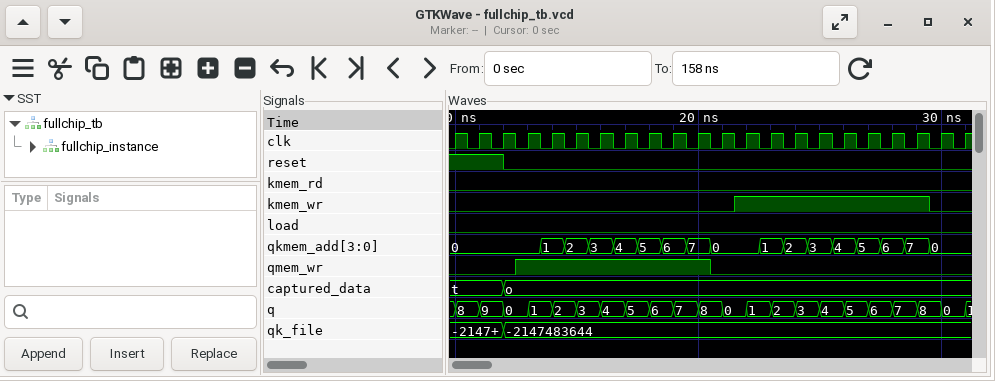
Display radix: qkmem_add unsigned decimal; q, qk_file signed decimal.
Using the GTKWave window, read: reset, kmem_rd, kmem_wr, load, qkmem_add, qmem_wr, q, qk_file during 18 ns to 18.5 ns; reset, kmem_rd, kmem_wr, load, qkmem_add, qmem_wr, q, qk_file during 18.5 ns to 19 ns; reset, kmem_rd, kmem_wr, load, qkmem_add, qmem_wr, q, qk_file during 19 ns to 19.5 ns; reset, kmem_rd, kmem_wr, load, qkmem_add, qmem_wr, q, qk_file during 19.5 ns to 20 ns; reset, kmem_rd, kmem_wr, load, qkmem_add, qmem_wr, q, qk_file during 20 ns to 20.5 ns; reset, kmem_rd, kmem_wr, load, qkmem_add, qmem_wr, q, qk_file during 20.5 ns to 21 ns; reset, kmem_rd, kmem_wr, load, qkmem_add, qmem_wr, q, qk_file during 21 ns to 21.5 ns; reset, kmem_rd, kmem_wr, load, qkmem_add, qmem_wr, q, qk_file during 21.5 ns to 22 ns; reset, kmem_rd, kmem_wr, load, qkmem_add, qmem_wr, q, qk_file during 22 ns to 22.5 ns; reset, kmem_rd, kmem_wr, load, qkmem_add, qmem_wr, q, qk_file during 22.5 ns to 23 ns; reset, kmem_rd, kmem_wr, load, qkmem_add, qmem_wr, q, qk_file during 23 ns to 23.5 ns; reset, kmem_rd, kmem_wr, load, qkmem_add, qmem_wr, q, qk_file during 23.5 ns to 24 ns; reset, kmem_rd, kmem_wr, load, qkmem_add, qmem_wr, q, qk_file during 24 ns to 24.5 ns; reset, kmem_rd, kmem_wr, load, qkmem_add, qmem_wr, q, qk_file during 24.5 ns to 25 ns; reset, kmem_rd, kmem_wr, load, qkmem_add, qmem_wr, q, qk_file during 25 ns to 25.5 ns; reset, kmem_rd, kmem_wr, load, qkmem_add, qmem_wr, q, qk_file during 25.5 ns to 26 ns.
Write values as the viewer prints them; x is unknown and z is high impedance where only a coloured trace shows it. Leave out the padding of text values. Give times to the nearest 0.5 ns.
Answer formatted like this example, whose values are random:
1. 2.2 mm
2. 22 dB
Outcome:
1. reset=0, kmem_rd=0, kmem_wr=0, load=0, qkmem_add=5, qmem_wr=1, q=6, qk_file=-2147483644
2. reset=0, kmem_rd=0, kmem_wr=0, load=0, qkmem_add=6, qmem_wr=1, q=6, qk_file=-2147483644
3. reset=0, kmem_rd=0, kmem_wr=0, load=0, qkmem_add=6, qmem_wr=1, q=7, qk_file=-2147483644
4. reset=0, kmem_rd=0, kmem_wr=0, load=0, qkmem_add=7, qmem_wr=1, q=7, qk_file=-2147483644
5. reset=0, kmem_rd=0, kmem_wr=0, load=0, qkmem_add=7, qmem_wr=1, q=8, qk_file=-2147483644
6. reset=0, kmem_rd=0, kmem_wr=0, load=0, qkmem_add=0, qmem_wr=0, q=8, qk_file=-2147483644
7. reset=0, kmem_rd=0, kmem_wr=0, load=0, qkmem_add=0, qmem_wr=0, q=0, qk_file=-2147483644
8. reset=0, kmem_rd=0, kmem_wr=1, load=0, qkmem_add=0, qmem_wr=0, q=0, qk_file=-2147483644
9. reset=0, kmem_rd=0, kmem_wr=1, load=0, qkmem_add=0, qmem_wr=0, q=1, qk_file=-2147483644
10. reset=0, kmem_rd=0, kmem_wr=1, load=0, qkmem_add=1, qmem_wr=0, q=1, qk_file=-2147483644
11. reset=0, kmem_rd=0, kmem_wr=1, load=0, qkmem_add=1, qmem_wr=0, q=2, qk_file=-2147483644
12. reset=0, kmem_rd=0, kmem_wr=1, load=0, qkmem_add=2, qmem_wr=0, q=2, qk_file=-2147483644
13. reset=0, kmem_rd=0, kmem_wr=1, load=0, qkmem_add=2, qmem_wr=0, q=3, qk_file=-2147483644
14. reset=0, kmem_rd=0, kmem_wr=1, load=0, qkmem_add=3, qmem_wr=0, q=3, qk_file=-2147483644
15. reset=0, kmem_rd=0, kmem_wr=1, load=0, qkmem_add=3, qmem_wr=0, q=4, qk_file=-2147483644
16. reset=0, kmem_rd=0, kmem_wr=1, load=0, qkmem_add=4, qmem_wr=0, q=4, qk_file=-2147483644
